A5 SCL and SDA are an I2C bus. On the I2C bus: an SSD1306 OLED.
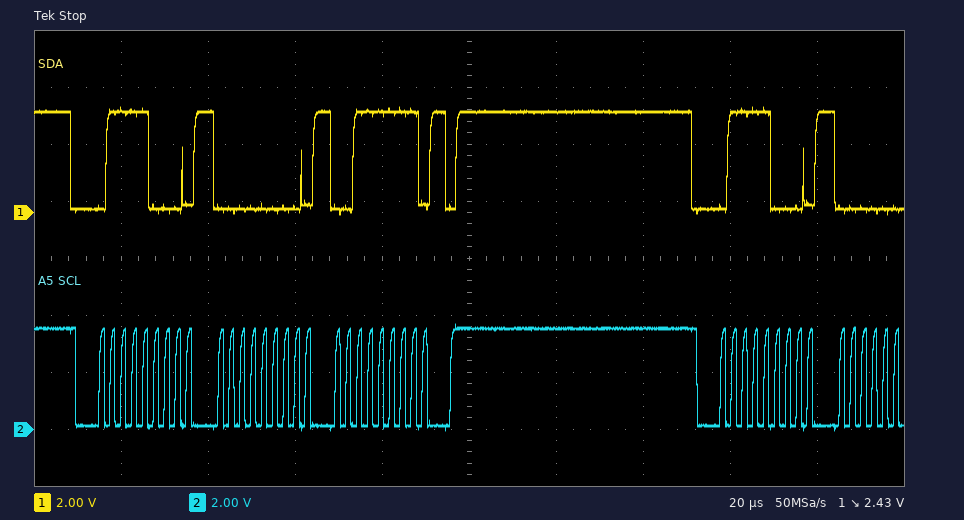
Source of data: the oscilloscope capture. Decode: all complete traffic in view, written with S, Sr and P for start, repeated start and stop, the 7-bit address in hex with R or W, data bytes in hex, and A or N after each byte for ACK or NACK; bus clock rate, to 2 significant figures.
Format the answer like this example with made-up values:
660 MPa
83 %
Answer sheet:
S 3CW A 00 A 3F A P S 3CW A
400 kHz
